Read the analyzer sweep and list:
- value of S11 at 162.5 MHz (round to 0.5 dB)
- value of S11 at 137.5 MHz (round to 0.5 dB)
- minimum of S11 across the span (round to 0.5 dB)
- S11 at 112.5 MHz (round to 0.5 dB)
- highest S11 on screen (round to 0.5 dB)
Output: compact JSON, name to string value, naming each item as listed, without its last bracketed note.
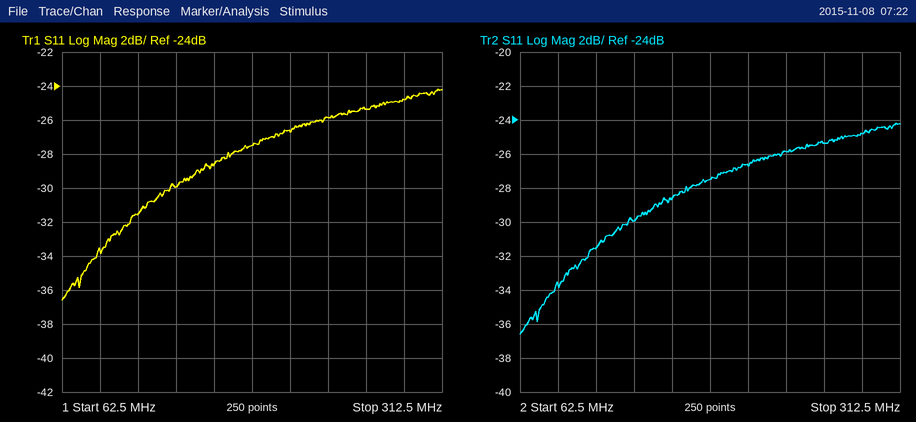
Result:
{"value of S11 at 162.5 MHz": "-28.5 dB", "value of S11 at 137.5 MHz": "-30.0 dB", "minimum of S11 across the span": "-36.5 dB", "S11 at 112.5 MHz": "-31.5 dB", "highest S11 on screen": "-24.0 dB"}
